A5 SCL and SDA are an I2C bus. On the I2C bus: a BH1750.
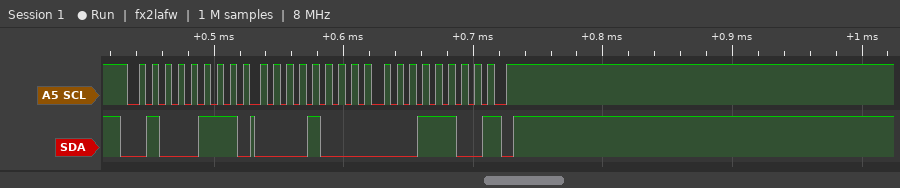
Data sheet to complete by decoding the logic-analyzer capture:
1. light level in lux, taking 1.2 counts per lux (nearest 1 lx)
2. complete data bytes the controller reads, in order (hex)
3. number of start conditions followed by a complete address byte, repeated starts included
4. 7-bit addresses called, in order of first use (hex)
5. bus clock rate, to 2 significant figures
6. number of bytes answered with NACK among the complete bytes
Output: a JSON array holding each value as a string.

["1730 lx", "08 1C", "1", "0x23", "100 kHz", "1"]
